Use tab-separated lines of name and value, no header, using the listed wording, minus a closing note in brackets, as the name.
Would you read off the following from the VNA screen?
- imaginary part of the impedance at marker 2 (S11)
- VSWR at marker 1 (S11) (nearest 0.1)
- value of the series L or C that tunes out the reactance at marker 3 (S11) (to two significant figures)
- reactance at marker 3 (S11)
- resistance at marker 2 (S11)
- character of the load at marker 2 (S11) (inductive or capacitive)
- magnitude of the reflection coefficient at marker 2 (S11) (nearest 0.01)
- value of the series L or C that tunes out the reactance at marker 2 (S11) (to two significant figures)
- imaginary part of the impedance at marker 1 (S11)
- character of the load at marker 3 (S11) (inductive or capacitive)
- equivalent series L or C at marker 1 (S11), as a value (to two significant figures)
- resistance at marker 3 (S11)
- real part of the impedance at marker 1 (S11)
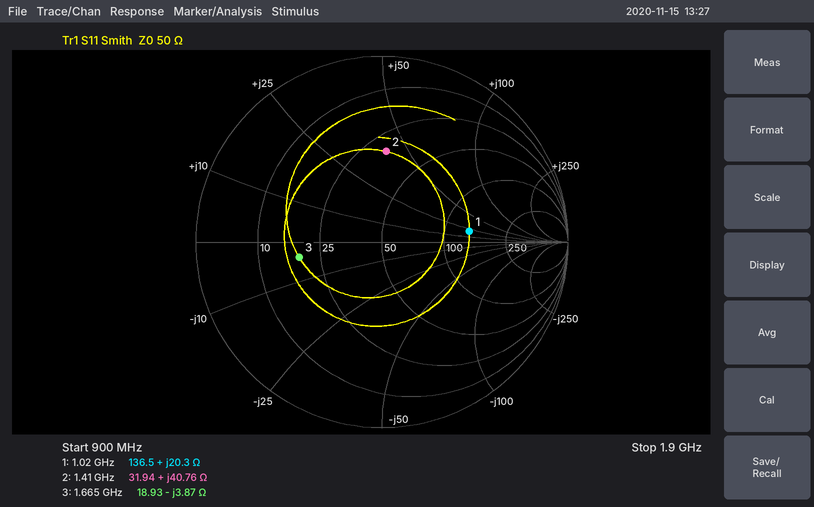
imaginary part of the impedance at marker 2	+40.76 Ω
VSWR at marker 1 (S11)	2.8
value of the series L or C that tunes out the reactance at marker 3 (S11)	370 pH
reactance at marker 3	-3.87 Ω
resistance at marker 2	31.94 Ω
character of the load at marker 2 (S11)	inductive
magnitude of the reflection coefficient at marker 2 (S11)	0.49
value of the series L or C that tunes out the reactance at marker 2 (S11)	2.8 pF
imaginary part of the impedance at marker 1	+20.3 Ω
character of the load at marker 3 (S11)	capacitive
equivalent series L or C at marker 1 (S11), as a value	3.2 nH
resistance at marker 3	18.93 Ω
real part of the impedance at marker 1	136.5 Ω
